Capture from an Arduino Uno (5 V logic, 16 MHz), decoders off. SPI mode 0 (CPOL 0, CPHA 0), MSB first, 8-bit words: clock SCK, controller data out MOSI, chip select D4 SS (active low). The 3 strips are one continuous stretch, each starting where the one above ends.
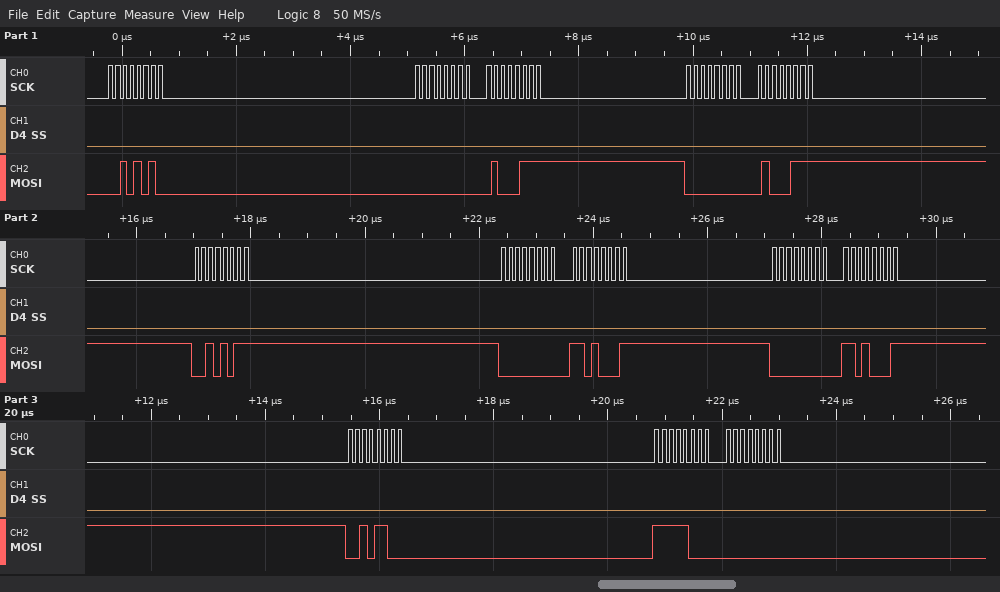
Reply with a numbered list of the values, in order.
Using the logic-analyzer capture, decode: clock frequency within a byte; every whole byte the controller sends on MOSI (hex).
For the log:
1. 8 MHz
2. 2A 00 47 00 47 2B 00 D1 00 D1 2C F8 00
